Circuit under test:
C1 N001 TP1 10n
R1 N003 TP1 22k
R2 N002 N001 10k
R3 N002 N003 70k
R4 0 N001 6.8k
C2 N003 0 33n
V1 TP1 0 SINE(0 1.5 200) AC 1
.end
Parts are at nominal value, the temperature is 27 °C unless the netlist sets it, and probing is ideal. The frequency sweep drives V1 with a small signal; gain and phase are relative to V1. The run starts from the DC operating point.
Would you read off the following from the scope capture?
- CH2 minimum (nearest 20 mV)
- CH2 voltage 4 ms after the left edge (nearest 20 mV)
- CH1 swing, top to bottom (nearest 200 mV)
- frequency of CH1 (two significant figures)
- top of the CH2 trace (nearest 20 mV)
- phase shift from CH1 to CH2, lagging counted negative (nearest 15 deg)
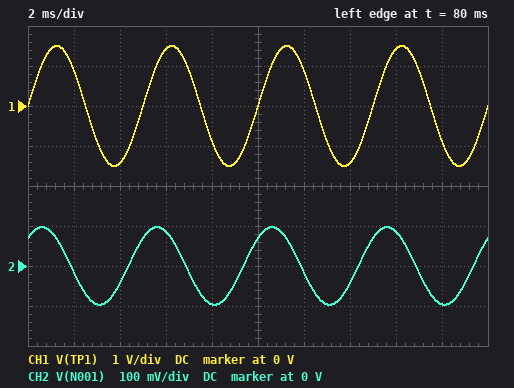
-100 mV
-40 mV
3.0 V
200 Hz
100 mV
45 deg
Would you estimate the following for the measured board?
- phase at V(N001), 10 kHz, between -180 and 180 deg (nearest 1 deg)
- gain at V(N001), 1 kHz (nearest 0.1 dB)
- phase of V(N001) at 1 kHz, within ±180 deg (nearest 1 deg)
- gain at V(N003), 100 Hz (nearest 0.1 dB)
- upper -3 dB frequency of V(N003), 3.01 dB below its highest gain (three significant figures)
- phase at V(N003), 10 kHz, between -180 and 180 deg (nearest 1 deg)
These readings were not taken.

14 deg
-9.1 dB
68 deg
-2.5 dB
276 Hz
-85 deg
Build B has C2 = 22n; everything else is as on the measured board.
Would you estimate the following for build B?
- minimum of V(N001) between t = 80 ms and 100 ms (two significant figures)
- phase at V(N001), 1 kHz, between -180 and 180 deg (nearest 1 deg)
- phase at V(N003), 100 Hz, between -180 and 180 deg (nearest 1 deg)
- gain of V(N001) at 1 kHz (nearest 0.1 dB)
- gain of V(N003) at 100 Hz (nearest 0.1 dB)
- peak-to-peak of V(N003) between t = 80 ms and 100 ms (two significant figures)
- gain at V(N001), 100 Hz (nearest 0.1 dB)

-110 mV
67 deg
-13 deg
-9.2 dB
-2.2 dB
2.2 V
-23.8 dB
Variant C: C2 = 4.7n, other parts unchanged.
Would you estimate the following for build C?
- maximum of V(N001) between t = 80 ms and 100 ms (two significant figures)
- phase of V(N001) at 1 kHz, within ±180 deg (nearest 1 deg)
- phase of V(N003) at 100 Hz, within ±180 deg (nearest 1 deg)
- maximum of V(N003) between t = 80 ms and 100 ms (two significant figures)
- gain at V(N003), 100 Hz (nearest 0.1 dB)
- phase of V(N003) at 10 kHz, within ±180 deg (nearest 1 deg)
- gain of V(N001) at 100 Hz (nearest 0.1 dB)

140 mV
60 deg
-2 deg
1.2 V
-2.0 dB
-76 deg
-22.8 dB
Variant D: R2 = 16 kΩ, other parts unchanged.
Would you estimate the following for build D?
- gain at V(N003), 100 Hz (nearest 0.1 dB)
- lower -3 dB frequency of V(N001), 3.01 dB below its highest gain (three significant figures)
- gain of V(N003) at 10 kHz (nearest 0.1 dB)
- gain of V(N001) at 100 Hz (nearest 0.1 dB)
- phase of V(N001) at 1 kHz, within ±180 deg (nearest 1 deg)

-2.4 dB
2.56 kHz
-31.3 dB
-25.0 dB
68 deg
